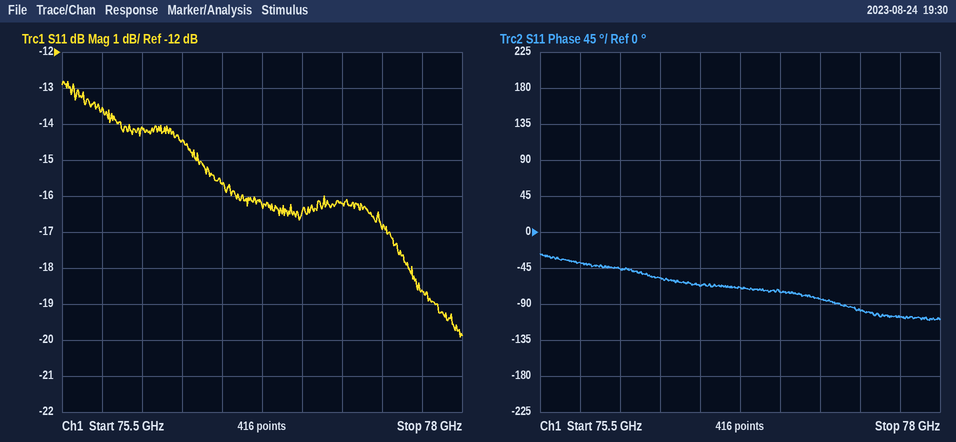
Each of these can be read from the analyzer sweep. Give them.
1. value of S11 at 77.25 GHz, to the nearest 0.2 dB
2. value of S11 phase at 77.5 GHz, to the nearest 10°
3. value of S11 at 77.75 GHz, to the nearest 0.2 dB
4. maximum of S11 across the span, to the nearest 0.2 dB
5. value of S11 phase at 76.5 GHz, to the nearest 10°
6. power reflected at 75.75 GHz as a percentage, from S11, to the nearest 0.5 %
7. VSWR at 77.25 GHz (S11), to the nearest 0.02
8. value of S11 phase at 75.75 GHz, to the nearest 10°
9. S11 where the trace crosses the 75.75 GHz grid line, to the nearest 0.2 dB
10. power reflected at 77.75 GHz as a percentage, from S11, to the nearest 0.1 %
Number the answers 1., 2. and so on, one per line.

1. -16.2 dB
2. -100°
3. -18.6 dB
4. -12.8 dB
5. -70°
6. 4.5 %
7. 1.36
8. -40°
9. -13.6 dB
10. 1.4 %
